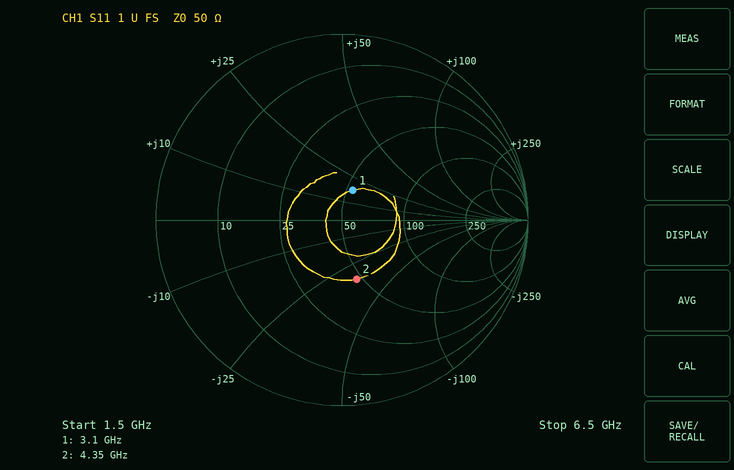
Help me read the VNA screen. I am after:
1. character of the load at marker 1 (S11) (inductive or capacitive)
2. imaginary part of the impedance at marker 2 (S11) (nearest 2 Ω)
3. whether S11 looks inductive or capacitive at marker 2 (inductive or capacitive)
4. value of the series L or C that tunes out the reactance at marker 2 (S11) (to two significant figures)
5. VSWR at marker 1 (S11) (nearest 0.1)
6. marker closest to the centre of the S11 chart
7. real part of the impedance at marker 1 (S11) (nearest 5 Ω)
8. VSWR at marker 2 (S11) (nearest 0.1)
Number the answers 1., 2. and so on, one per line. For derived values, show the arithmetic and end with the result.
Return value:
1. inductive
2. -34 Ω
3. capacitive
4. L = 34 Ω/(2π × 4.35 GHz) ≈ 1.2 nH
5. 1.4
6. marker 1
7. 55 Ω
8. 2.0
